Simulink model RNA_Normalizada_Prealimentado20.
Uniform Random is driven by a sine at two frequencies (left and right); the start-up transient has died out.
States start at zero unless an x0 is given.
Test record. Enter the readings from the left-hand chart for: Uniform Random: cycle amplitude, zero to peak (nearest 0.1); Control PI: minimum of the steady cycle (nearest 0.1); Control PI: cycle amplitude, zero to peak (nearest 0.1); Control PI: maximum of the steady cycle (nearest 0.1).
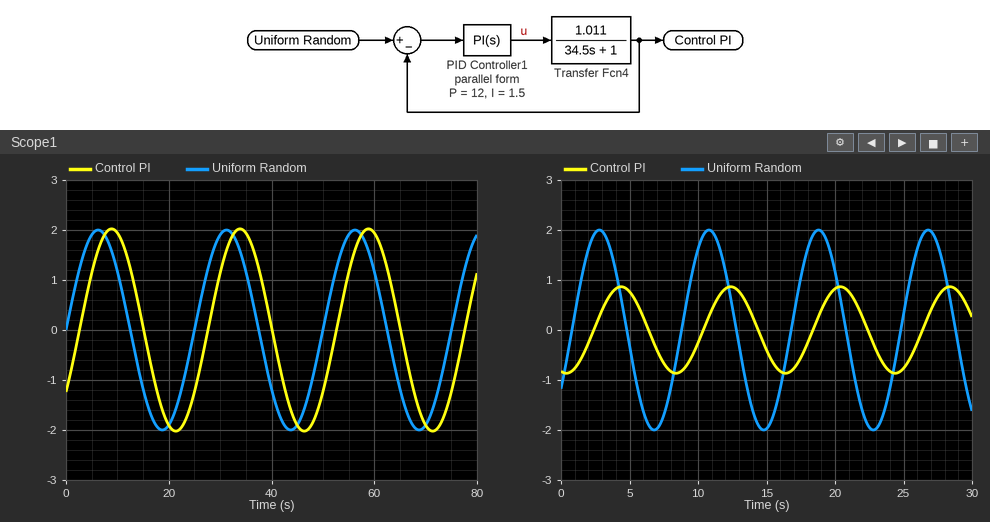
2.0
-2.0
2.0
2.0
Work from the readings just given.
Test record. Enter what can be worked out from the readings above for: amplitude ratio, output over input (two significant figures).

1.0
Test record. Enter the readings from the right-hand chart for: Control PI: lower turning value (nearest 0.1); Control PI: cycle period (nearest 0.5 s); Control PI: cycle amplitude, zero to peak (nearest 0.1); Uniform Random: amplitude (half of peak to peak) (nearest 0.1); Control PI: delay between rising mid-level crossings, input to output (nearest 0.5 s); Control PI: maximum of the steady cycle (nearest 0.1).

-0.9
8.0 s
0.9
2.0
1.5 s
0.9
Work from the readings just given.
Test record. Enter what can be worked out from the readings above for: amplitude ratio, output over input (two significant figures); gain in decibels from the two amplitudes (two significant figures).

0.45
-6.9 dB
